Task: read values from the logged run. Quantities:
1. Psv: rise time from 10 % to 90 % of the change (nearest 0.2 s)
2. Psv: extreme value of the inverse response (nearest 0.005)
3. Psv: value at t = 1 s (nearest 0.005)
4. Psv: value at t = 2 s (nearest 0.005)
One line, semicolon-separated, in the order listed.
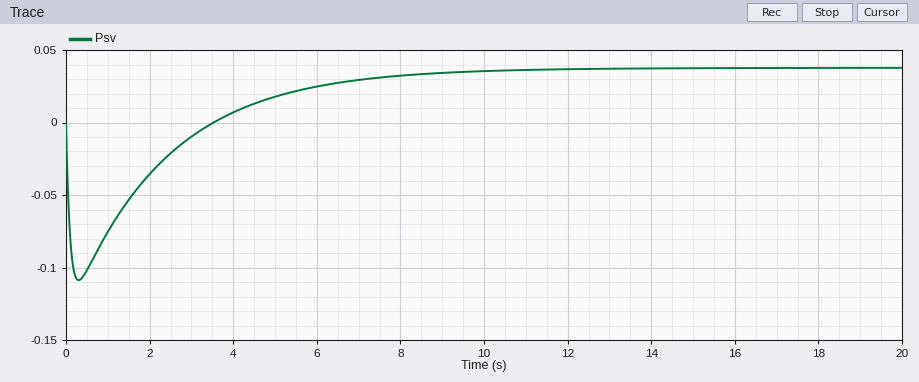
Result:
5.0 s; -0.110; -0.075; -0.035
